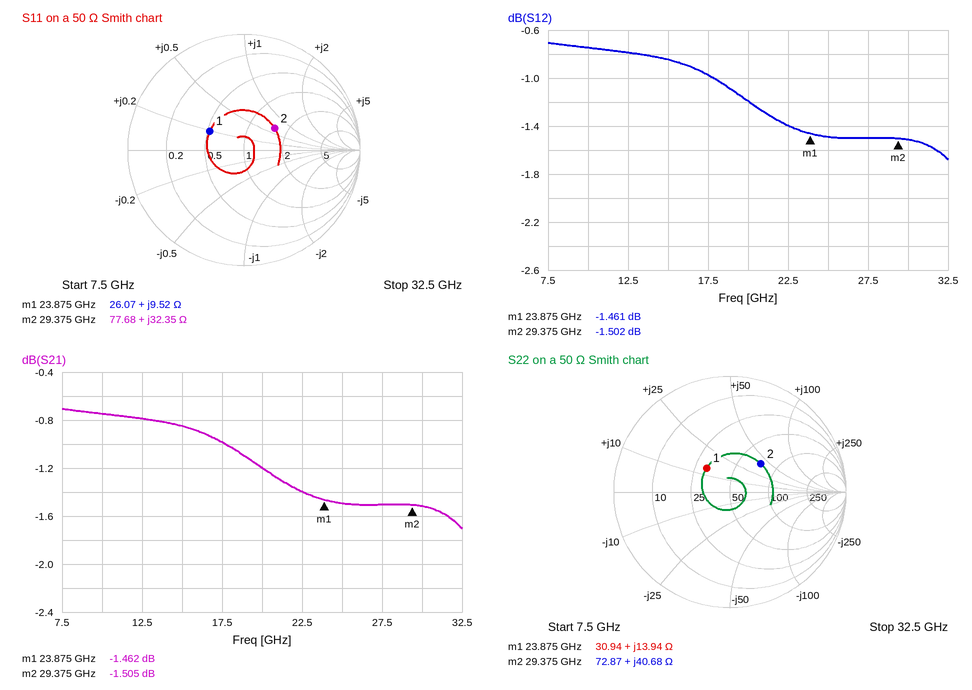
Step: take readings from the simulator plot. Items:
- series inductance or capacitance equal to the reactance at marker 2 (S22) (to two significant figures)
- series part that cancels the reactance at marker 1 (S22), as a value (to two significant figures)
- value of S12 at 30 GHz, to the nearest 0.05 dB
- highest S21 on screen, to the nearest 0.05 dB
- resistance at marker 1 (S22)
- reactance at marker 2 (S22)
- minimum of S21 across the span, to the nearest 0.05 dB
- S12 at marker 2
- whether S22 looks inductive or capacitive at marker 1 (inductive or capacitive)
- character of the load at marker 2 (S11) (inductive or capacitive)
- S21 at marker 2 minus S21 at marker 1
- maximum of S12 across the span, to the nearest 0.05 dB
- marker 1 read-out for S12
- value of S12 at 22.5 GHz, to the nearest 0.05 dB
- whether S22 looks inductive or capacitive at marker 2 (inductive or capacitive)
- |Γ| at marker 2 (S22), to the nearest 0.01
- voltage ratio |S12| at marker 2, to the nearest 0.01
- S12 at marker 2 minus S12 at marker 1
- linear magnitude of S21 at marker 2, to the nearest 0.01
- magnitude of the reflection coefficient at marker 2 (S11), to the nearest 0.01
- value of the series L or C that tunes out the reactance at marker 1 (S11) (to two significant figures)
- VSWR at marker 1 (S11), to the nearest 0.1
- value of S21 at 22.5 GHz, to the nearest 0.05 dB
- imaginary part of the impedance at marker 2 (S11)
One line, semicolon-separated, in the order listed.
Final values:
220 pH; 480 fF; -1.50 dB; -0.70 dB; 30.94 Ω; +40.68 Ω; -1.70 dB; -1.502 dB; inductive; inductive; -0.043 dB; -0.70 dB; -1.461 dB; -1.40 dB; inductive; 0.36; 0.84; -0.041 dB; 0.84; 0.32; 700 fF; 2.0; -1.40 dB; +32.35 Ω
